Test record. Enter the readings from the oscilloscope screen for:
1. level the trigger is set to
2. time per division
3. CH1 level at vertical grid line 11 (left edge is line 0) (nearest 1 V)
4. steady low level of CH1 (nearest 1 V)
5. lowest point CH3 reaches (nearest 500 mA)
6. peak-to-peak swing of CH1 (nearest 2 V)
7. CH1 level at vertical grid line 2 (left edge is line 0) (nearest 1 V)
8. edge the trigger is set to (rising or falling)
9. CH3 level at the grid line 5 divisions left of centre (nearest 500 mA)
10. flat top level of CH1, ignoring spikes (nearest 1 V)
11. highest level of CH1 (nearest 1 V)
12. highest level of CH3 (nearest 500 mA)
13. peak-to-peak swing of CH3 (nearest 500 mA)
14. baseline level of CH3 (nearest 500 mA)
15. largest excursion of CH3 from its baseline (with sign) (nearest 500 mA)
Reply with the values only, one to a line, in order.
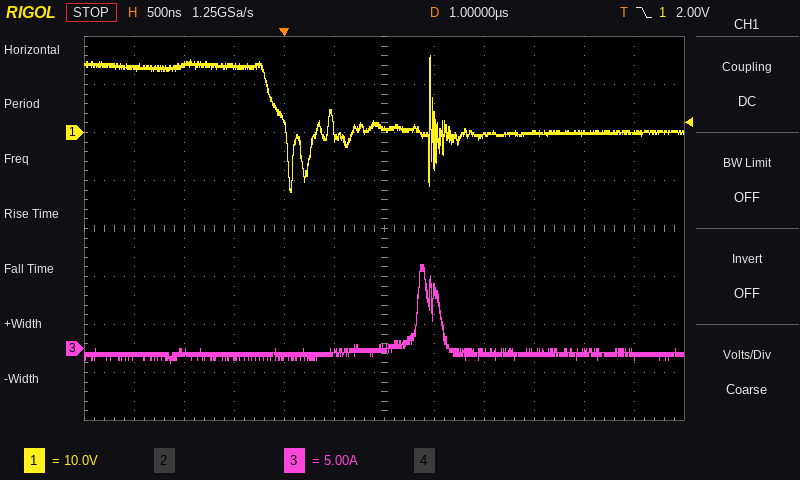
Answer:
2.00 V
500 ns
0 V
0 V
-1.5 A
28 V
14 V
falling
-1.0 A
14 V
16 V
9.0 A
10.5 A
-500 mA
+9.5 A
